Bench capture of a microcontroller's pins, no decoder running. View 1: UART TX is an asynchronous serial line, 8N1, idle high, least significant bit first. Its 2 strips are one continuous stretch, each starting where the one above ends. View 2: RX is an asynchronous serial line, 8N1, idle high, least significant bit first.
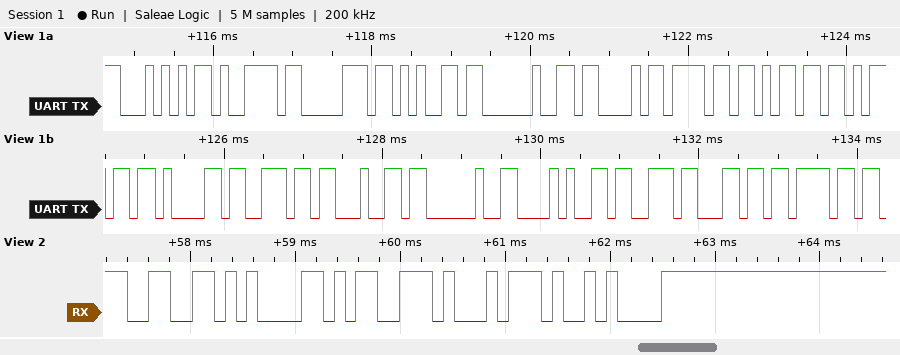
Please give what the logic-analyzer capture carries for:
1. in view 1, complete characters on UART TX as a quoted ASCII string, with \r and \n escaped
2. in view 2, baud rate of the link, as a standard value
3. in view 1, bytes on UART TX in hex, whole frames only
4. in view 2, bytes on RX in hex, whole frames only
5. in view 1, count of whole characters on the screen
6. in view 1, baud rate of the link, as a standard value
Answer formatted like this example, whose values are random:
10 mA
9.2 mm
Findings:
"Type Command (slo"
9600 baud
54 79 70 65 20 43 6F 6D 6D 61 6E 64 20 28 73 6C 6F
66 61 73 74 0A
17
9600 baud
